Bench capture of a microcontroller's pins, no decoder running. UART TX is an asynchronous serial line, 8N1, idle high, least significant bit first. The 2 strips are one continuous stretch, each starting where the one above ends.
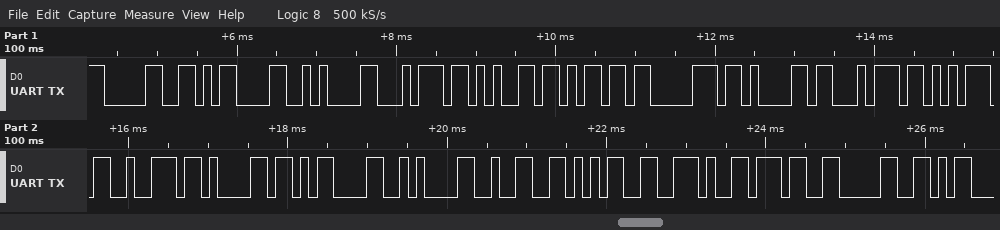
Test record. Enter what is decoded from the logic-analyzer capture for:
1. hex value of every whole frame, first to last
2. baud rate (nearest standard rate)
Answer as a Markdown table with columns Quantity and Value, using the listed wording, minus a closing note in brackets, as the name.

| Quantity | Value |
|---|---|
| hex value of every whole frame, first to last | 0x30 0x0D 0x0A 0x74 0x65 0x6D 0x70 0x61 0x74 0x75 0x72 0x61 0x0D 0x0A 0x32 0x35 0x2E 0x37 0x30 |
| baud rate | 9600 baud |
